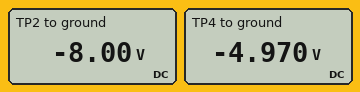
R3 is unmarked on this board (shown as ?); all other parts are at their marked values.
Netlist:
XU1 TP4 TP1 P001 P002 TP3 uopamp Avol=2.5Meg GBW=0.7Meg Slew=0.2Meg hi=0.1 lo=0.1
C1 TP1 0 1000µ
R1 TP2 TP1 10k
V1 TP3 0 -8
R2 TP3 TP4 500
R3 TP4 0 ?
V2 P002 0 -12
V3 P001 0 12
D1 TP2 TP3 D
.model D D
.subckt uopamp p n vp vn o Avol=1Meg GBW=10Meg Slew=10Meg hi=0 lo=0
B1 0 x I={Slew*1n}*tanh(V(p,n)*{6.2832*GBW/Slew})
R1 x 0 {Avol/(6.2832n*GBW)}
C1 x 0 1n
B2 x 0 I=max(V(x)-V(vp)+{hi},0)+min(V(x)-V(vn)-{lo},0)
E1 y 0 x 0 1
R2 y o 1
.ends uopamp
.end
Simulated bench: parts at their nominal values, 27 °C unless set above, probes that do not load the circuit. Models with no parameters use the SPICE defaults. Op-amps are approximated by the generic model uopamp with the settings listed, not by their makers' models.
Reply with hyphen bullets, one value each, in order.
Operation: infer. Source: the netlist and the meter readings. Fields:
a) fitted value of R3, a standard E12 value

- 820 Ω
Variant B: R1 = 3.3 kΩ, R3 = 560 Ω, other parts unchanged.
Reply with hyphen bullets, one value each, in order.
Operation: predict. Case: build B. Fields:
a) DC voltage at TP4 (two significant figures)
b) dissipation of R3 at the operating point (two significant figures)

- -4.2 V
- 32 mW
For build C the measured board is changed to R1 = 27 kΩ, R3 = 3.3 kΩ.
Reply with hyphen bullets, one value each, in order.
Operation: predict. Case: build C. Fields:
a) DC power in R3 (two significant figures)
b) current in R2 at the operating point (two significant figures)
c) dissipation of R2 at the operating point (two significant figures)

- 15 mW
- 2.1 mA
- 2.2 mW
